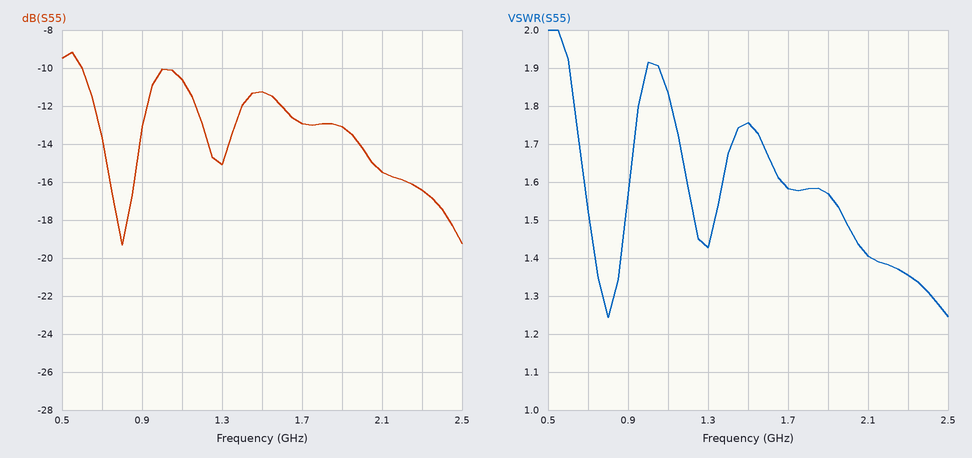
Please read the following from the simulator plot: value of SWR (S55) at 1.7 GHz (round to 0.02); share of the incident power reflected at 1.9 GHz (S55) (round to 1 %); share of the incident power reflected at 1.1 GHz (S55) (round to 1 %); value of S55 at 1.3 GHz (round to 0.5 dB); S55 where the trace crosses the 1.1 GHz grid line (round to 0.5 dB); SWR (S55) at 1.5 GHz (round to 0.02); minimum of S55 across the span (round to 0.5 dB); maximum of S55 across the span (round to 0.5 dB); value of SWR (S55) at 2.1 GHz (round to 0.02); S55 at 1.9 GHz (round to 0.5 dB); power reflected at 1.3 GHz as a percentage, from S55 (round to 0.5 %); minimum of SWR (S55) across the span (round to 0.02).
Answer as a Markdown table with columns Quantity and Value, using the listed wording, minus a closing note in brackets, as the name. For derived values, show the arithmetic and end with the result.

| Quantity | Value |
|---|---|
| value of SWR (S55) at 1.7 GHz | 1.58 |
| share of the incident power reflected at 1.9 GHz (S55) | 10^(-13/10) ≈ 5 % |
| share of the incident power reflected at 1.1 GHz (S55) | 10^(-10.5/10) ≈ 9 % |
| value of S55 at 1.3 GHz | -15.0 dB |
| S55 where the trace crosses the 1.1 GHz grid line | -10.5 dB |
| SWR (S55) at 1.5 GHz | 1.76 |
| minimum of S55 across the span | -19.5 dB |
| maximum of S55 across the span | -9.0 dB |
| value of SWR (S55) at 2.1 GHz | 1.40 |
| S55 at 1.9 GHz | -13.0 dB |
| power reflected at 1.3 GHz as a percentage, from S55 | 10^(-15/10) ≈ 3.16 %, so 3.0 % to the nearest 0.5 % |
| minimum of SWR (S55) across the span | 1.24 |
